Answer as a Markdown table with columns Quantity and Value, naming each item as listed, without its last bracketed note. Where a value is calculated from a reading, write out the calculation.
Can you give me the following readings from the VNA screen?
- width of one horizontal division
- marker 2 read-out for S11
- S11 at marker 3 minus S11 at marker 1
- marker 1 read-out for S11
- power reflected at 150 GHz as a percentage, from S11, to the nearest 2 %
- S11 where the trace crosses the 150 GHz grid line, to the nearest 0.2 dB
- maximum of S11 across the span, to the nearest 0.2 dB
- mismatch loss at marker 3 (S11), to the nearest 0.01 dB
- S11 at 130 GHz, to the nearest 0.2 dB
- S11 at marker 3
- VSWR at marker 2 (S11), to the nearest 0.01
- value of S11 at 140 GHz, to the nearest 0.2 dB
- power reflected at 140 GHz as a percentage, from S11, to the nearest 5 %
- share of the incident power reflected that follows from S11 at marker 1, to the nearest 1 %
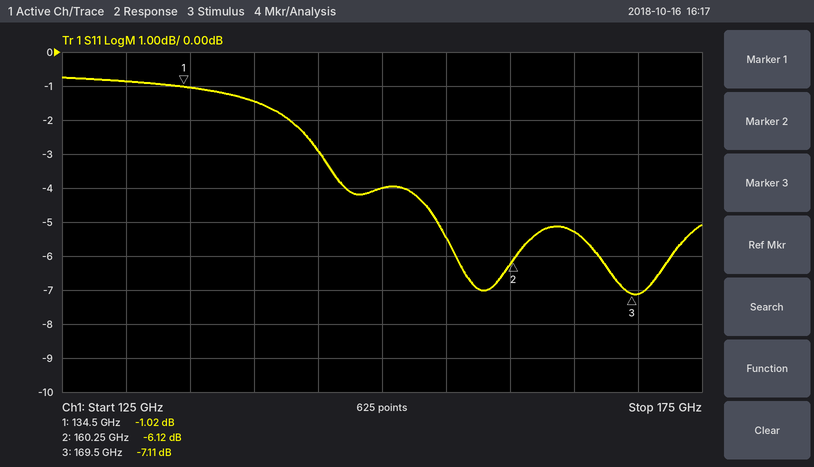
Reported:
| Quantity | Value |
|---|---|
| width of one horizontal division | 5 GHz |
| marker 2 read-out for S11 | -6.12 dB |
| S11 at marker 3 minus S11 at marker 1 | -7.11 − (-1.02) = -6.09 dB |
| marker 1 read-out for S11 | -1.02 dB |
| power reflected at 150 GHz as a percentage, from S11, to the nearest 2 % | 10^(-4/10) ≈ 40 % |
| S11 where the trace crosses the 150 GHz grid line, to the nearest 0.2 dB | -4.0 dB |
| maximum of S11 across the span, to the nearest 0.2 dB | -0.8 dB |
| mismatch loss at marker 3 (S11), to the nearest 0.01 dB | −10 log10(1 − 10^(-7.11/10)) ≈ 0.94 dB |
| S11 at 130 GHz, to the nearest 0.2 dB | -0.8 dB |
| S11 at marker 3 | -7.11 dB |
| VSWR at marker 2 (S11), to the nearest 0.01 | (1 + 0.4943)/(1 − 0.4943) ≈ 2.95 |
| value of S11 at 140 GHz, to the nearest 0.2 dB | -1.4 dB |
| power reflected at 140 GHz as a percentage, from S11, to the nearest 5 % | 10^(-1.4/10) ≈ 72.4 %, so 70 % to the nearest 5 % |
| share of the incident power reflected that follows from S11 at marker 1, to the nearest 1 % | 10^(-1.02/10) ≈ 79 % |
